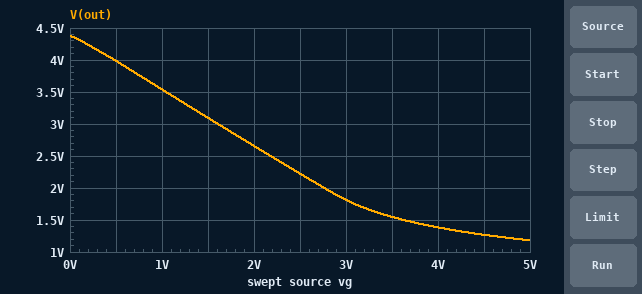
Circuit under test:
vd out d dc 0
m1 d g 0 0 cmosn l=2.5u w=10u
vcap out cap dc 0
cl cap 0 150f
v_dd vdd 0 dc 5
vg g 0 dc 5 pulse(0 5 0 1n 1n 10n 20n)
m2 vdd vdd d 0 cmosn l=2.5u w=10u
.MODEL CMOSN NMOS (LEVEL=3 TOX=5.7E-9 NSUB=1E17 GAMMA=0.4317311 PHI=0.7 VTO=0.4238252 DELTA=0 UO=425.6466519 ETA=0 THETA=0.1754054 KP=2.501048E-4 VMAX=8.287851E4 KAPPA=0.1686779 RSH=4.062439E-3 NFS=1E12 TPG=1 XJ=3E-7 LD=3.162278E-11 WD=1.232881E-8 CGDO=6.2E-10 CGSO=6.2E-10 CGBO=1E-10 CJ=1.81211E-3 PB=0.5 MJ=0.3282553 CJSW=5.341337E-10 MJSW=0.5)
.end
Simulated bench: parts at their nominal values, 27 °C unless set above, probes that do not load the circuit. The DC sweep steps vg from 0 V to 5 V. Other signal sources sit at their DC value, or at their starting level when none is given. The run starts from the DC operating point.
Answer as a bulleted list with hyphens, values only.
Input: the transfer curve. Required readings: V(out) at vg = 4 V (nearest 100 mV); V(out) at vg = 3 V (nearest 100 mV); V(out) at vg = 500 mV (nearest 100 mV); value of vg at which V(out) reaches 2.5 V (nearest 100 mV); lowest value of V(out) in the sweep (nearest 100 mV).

- 1.4 V
- 1.8 V
- 4.0 V
- 2.2 V
- 1.2 V
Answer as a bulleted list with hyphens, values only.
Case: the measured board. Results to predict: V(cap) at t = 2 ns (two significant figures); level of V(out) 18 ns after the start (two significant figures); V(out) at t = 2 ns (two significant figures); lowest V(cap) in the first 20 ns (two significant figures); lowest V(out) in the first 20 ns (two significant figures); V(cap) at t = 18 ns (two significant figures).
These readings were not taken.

- 1.2 V
- 4.0 V
- 1.2 V
- 1.1 V
- 1.1 V
- 4.0 V
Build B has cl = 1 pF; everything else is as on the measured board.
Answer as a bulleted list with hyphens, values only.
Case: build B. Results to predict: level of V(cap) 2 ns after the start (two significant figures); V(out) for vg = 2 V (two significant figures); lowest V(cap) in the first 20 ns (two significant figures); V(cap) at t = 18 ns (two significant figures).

- 1.5 V
- 2.7 V
- 1.2 V
- 3.7 V
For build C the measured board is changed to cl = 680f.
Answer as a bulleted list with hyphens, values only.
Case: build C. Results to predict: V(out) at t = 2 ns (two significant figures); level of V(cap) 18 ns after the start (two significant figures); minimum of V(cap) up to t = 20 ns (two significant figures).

- 1.3 V
- 3.8 V
- 1.2 V
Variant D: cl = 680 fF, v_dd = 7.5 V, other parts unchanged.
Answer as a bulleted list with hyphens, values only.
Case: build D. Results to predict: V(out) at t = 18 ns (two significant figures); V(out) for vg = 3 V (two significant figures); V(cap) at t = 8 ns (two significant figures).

- 6.1 V
- 4.1 V
- 2.5 V
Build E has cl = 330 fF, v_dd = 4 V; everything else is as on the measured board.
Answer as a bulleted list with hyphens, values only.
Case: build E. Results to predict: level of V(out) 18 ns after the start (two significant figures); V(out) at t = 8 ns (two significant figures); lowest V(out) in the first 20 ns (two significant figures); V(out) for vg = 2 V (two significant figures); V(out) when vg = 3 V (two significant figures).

- 3.0 V
- 800 mV
- 750 mV
- 1.8 V
- 1.1 V
